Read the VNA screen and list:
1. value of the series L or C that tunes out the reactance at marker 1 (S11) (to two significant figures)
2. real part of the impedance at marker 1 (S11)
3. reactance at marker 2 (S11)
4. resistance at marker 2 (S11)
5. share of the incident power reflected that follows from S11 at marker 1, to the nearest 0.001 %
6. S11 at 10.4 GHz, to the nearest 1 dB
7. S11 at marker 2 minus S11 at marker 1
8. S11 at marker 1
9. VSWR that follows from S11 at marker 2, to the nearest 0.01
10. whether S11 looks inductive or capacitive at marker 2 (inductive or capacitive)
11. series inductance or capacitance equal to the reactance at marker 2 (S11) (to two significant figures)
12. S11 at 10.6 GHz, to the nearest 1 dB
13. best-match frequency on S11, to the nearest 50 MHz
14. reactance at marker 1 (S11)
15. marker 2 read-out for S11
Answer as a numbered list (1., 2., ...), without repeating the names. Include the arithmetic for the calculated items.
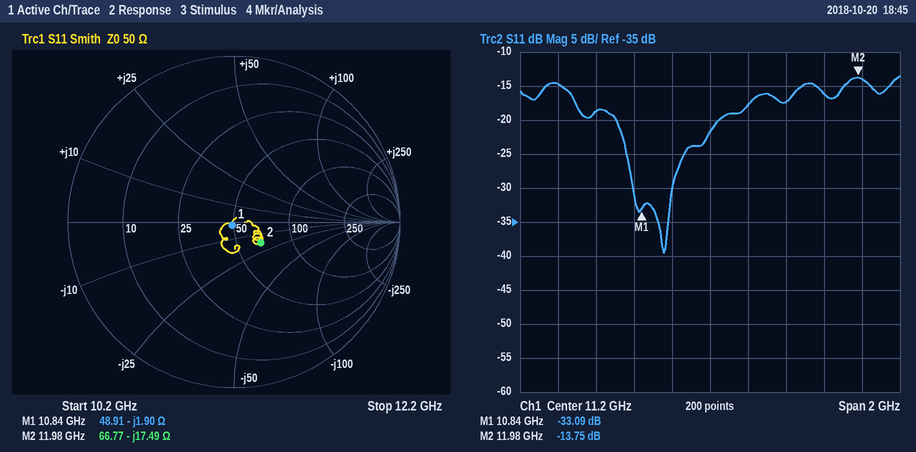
1. L = 1.9 Ω/(2π × 10.84 GHz) ≈ 28 pH
2. 48.91 Ω
3. -17.49 Ω
4. 66.77 Ω
5. 10^(-33.09/10) ≈ 0.049 %
6. -15 dB
7. -13.75 − (-33.09) = 19.34 dB
8. -33.09 dB
9. (1 + 0.2054)/(1 − 0.2054) ≈ 1.52
10. capacitive
11. C = 1/(2π × 11.98 GHz × 17.49 Ω) ≈ 760 fF
12. -19 dB
13. 10.95 GHz
14. -1.90 Ω
15. -13.75 dB
